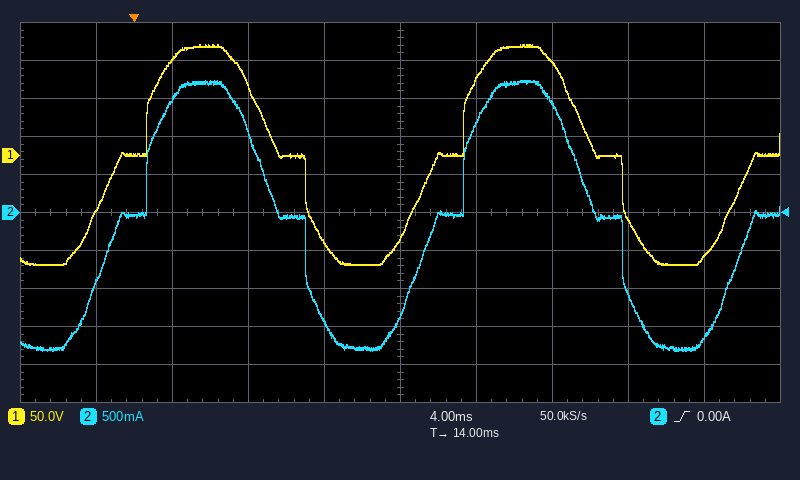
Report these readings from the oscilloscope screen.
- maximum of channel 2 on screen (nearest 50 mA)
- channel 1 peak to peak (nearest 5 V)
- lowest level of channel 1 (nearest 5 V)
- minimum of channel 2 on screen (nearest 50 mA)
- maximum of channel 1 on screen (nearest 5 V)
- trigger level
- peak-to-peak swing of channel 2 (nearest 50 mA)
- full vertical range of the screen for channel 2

1.75 A
290 V
-145 V
-1.80 A
145 V
0.00 A
3.55 A
5 A
